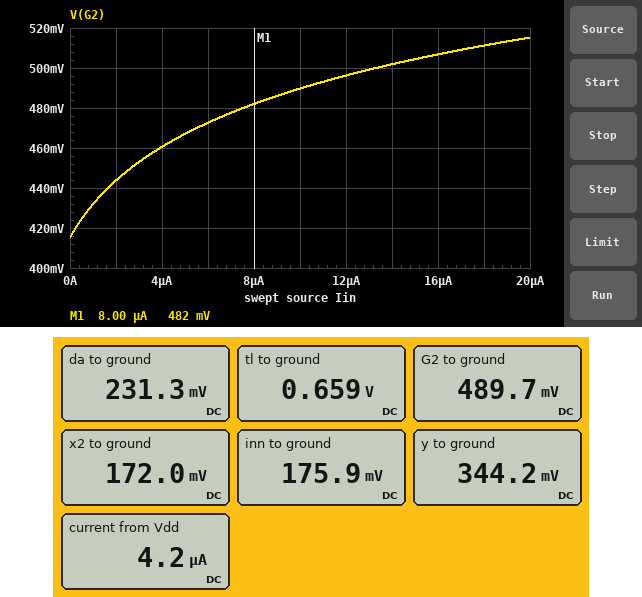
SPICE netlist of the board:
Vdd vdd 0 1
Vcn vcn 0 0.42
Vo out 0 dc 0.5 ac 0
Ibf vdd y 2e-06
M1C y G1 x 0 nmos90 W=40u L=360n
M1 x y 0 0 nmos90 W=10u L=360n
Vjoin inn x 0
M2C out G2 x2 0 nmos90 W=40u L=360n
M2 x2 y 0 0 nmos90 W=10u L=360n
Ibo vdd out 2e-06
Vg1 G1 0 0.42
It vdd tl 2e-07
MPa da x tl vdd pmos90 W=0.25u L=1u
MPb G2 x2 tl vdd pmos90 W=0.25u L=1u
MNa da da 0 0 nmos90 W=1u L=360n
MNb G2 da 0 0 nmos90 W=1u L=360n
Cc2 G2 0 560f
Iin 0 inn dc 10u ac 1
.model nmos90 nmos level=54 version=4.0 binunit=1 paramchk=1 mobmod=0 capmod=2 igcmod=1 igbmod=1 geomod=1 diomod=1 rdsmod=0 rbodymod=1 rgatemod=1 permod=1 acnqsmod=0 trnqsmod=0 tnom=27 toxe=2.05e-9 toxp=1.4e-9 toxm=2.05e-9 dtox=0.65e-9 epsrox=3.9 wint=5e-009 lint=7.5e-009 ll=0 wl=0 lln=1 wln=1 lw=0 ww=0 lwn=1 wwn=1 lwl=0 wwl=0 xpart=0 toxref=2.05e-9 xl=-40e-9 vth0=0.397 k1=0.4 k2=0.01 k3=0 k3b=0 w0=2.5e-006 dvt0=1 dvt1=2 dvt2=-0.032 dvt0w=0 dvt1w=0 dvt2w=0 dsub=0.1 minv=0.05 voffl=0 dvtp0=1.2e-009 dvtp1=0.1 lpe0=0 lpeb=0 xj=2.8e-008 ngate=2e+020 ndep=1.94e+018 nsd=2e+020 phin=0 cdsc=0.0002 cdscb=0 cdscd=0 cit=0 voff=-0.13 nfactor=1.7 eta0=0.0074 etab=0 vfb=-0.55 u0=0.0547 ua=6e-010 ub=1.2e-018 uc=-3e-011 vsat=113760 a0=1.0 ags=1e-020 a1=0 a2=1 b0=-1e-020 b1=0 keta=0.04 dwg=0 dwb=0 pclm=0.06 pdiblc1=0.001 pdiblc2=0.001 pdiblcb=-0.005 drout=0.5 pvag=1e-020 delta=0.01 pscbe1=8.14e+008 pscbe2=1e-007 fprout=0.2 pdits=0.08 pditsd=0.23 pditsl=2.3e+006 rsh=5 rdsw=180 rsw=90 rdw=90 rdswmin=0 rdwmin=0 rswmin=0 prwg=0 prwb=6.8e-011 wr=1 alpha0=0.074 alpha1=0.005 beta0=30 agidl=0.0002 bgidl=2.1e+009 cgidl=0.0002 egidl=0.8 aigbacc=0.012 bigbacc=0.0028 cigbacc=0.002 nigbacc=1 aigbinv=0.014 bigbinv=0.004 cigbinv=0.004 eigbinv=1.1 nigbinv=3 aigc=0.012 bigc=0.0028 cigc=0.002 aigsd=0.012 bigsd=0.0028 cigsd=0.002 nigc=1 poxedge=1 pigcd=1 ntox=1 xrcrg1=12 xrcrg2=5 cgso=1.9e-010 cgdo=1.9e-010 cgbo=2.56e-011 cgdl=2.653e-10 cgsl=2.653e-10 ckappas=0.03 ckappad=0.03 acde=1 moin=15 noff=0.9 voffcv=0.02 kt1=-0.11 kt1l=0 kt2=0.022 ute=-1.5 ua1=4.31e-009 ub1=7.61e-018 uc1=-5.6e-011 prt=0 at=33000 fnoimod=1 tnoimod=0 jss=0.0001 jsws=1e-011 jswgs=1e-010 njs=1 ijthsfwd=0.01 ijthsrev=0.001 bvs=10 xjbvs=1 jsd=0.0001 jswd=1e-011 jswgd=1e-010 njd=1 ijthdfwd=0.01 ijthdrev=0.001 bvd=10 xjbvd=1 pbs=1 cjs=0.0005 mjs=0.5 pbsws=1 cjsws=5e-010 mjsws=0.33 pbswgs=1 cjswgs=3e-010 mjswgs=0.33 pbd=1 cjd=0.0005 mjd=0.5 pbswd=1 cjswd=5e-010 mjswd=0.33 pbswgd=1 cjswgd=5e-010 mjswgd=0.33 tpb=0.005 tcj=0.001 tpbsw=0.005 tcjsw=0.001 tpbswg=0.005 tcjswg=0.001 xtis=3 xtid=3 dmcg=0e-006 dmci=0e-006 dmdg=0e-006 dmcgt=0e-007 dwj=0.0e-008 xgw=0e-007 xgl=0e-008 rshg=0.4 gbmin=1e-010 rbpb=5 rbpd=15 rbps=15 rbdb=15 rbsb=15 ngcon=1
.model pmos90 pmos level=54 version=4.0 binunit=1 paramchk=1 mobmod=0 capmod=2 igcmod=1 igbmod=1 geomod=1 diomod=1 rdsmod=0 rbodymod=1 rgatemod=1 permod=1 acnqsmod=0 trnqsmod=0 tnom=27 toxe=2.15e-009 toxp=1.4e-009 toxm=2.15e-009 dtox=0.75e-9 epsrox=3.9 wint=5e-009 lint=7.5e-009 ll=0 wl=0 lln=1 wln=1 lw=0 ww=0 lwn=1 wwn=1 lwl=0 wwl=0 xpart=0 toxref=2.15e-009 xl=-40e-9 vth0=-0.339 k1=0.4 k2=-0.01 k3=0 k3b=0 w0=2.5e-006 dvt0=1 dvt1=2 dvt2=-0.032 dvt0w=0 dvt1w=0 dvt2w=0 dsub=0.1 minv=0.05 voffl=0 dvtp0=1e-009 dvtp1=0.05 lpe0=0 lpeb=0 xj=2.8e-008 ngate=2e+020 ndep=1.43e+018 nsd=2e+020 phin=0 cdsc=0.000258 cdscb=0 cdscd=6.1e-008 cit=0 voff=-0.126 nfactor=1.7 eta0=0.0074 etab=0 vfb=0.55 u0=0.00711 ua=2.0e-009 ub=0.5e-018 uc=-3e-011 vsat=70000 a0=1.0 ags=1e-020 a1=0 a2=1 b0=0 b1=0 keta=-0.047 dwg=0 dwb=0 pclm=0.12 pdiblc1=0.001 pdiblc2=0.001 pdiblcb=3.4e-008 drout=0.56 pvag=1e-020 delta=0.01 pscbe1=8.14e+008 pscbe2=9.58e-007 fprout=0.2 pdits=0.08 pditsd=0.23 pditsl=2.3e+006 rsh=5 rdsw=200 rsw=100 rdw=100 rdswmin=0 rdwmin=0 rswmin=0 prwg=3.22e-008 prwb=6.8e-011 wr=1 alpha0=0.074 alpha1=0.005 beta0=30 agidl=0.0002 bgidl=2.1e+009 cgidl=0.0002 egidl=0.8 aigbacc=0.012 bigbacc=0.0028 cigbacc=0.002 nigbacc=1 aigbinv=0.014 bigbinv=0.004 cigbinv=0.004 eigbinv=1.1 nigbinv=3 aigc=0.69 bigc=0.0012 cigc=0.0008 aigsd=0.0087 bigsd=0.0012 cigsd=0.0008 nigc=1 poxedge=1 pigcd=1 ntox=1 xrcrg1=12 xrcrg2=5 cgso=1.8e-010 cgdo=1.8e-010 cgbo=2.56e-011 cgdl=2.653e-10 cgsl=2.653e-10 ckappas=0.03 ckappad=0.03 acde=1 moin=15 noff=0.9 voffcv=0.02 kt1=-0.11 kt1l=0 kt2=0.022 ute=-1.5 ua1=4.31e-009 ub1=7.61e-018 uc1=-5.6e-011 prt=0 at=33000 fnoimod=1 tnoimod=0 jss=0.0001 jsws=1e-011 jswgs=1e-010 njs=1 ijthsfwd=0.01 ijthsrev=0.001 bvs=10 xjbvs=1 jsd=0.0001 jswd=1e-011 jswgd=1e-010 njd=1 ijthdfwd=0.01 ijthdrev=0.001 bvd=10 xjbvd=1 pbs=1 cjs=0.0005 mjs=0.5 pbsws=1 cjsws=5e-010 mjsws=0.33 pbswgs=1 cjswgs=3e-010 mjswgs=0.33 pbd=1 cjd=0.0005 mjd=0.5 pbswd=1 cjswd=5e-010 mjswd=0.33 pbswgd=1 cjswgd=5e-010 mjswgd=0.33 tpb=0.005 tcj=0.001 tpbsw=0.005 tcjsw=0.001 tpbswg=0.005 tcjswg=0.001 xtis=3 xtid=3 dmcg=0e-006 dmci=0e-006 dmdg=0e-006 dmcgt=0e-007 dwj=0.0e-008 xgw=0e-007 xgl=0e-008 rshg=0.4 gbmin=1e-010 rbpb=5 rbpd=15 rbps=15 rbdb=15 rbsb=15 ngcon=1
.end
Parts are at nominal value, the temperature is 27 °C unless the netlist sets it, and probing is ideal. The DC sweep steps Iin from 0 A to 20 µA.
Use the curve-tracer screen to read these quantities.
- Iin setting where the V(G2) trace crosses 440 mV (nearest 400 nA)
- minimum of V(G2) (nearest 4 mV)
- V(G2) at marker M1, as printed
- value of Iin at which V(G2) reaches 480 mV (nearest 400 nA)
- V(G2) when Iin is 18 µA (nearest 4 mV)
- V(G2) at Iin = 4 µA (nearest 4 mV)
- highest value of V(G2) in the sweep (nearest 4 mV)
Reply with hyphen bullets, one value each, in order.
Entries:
- 1.6 µA
- 416 mV
- 482 mV
- 7.6 µA
- 512 mV
- 460 mV
- 516 mV
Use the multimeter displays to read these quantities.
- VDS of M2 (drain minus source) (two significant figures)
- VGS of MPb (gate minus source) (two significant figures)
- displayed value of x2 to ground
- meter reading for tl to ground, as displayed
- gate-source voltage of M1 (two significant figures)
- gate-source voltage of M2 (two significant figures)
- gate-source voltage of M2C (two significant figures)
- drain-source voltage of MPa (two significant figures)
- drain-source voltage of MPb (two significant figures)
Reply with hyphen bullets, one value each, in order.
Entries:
- 170 mV
- -490 mV
- 172.0 mV
- 0.659 V
- 340 mV
- 340 mV
- 320 mV
- -430 mV
- -170 mV
